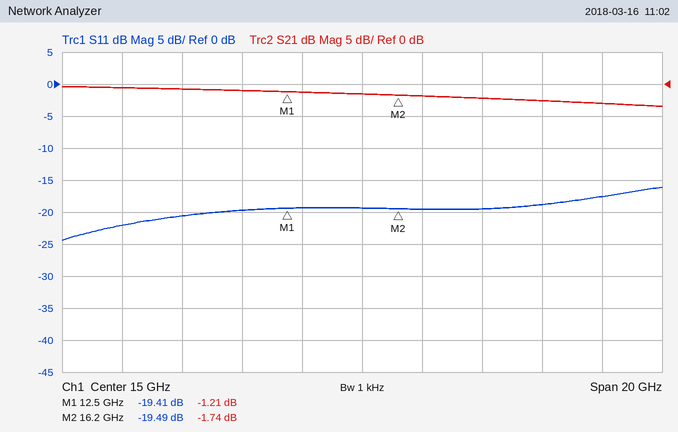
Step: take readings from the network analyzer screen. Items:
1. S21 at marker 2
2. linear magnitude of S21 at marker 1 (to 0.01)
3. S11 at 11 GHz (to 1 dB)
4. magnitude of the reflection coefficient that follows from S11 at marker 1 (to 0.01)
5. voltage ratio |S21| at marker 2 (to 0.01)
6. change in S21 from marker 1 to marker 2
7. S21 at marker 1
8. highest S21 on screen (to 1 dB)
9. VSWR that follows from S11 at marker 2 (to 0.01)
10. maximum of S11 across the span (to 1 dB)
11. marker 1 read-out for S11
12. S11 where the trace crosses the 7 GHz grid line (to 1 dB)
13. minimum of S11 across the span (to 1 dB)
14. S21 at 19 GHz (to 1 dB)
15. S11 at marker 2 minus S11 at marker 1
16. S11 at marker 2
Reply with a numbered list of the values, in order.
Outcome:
1. -1.74 dB
2. 0.87
3. -20 dB
4. 0.11
5. 0.82
6. -0.53 dB
7. -1.21 dB
8. 0 dB
9. 1.24
10. -16 dB
11. -19.41 dB
12. -22 dB
13. -24 dB
14. -2 dB
15. -0.08 dB
16. -19.49 dB
